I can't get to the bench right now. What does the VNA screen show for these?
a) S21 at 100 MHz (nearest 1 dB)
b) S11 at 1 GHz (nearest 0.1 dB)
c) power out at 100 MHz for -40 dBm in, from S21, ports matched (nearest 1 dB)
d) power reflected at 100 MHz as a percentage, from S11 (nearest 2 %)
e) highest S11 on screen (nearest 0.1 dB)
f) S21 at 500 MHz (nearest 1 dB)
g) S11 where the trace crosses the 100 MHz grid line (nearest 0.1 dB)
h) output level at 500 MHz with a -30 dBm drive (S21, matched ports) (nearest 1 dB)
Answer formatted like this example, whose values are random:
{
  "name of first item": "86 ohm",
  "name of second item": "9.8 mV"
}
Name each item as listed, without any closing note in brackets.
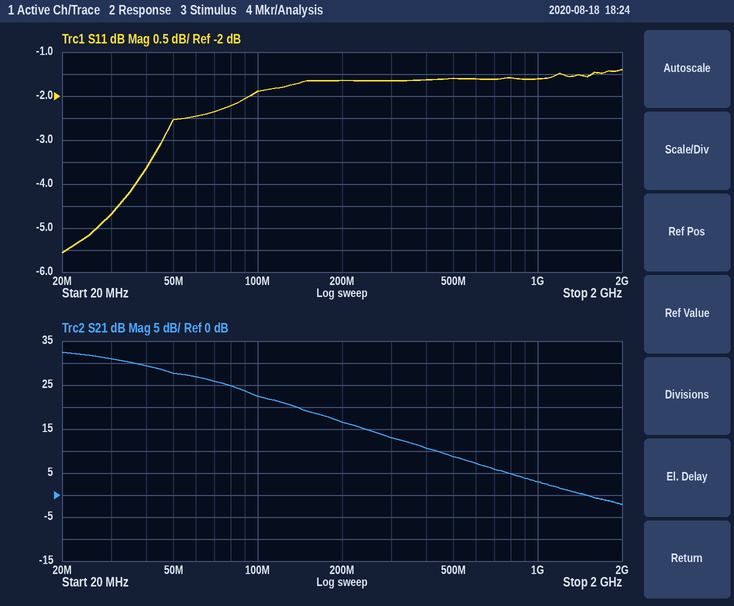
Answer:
{
  "S21 at 100 MHz": "22 dB",
  "S11 at 1 GHz": "-1.6 dB",
  "power out at 100 MHz for -40 dBm in, from S21, ports matched": "-18 dBm",
  "power reflected at 100 MHz as a percentage, from S11": "64 %",
  "highest S11 on screen": "-1.4 dB",
  "S21 at 500 MHz": "9 dB",
  "S11 where the trace crosses the 100 MHz grid line": "-1.9 dB",
  "output level at 500 MHz with a -30 dBm drive (S21, matched ports)": "-21 dBm"
}
